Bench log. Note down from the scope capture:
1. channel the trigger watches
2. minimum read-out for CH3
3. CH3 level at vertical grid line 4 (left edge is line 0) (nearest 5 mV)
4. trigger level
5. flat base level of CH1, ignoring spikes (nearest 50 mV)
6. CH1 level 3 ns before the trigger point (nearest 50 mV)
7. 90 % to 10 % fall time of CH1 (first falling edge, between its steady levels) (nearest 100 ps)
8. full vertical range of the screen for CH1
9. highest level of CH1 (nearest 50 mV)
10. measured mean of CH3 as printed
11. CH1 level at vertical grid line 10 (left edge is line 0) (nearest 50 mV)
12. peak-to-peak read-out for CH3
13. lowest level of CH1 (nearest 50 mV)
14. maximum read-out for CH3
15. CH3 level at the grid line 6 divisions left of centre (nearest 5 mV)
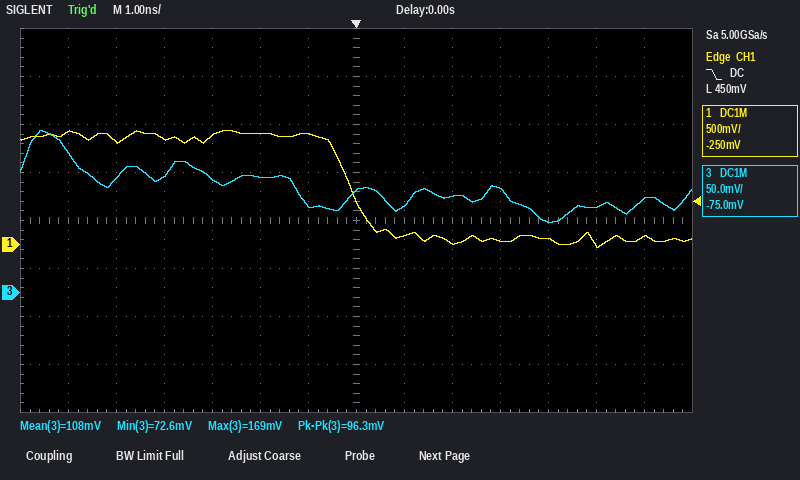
CH1
72.6 mV
120 mV
450 mV
50 mV
1.15 V
900 ps
4 V
1.20 V
108 mV
50 mV
96.3 mV
-50 mV
169 mV
145 mV
